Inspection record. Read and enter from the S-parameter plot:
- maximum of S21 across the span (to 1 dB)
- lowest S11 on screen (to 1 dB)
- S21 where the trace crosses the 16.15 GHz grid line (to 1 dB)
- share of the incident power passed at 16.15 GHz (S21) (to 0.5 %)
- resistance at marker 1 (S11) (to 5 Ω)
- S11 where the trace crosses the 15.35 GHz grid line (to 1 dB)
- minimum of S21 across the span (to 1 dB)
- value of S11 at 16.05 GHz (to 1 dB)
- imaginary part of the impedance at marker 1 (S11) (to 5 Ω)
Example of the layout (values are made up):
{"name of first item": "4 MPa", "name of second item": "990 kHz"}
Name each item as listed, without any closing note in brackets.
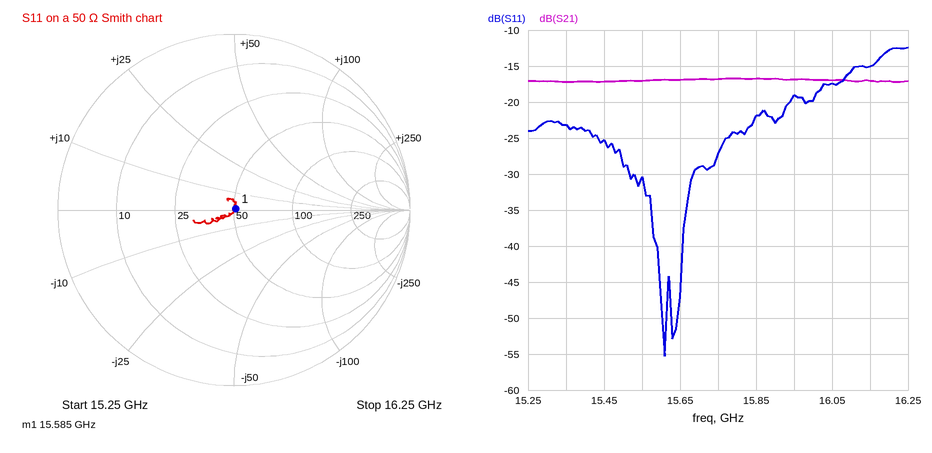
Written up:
{"maximum of S21 across the span": "-17 dB", "lowest S11 on screen": "-55 dB", "S21 where the trace crosses the 16.15 GHz grid line": "-17 dB", "share of the incident power passed at 16.15 GHz (S21)": "2.0 %", "resistance at marker 1 (S11)": "50 Ω", "S11 where the trace crosses the 15.35 GHz grid line": "-23 dB", "minimum of S21 across the span": "-17 dB", "value of S11 at 16.05 GHz": "-17 dB", "imaginary part of the impedance at marker 1 (S11)": "0 Ω"}
